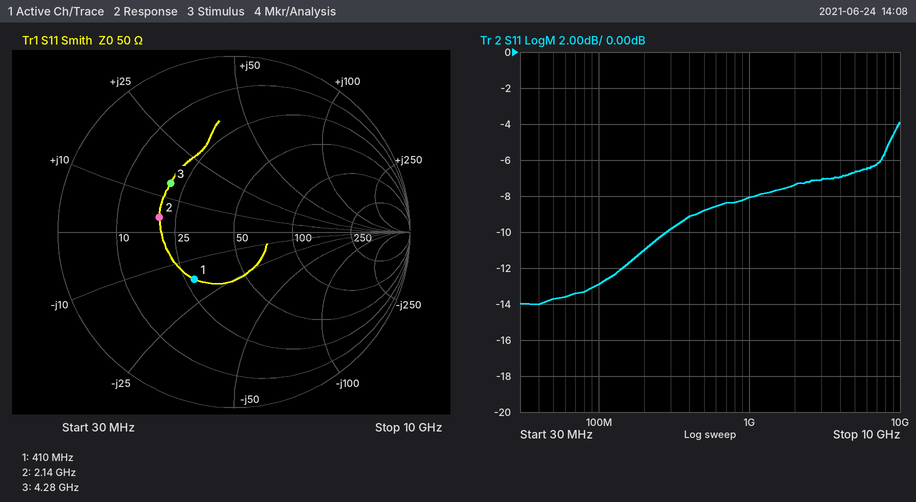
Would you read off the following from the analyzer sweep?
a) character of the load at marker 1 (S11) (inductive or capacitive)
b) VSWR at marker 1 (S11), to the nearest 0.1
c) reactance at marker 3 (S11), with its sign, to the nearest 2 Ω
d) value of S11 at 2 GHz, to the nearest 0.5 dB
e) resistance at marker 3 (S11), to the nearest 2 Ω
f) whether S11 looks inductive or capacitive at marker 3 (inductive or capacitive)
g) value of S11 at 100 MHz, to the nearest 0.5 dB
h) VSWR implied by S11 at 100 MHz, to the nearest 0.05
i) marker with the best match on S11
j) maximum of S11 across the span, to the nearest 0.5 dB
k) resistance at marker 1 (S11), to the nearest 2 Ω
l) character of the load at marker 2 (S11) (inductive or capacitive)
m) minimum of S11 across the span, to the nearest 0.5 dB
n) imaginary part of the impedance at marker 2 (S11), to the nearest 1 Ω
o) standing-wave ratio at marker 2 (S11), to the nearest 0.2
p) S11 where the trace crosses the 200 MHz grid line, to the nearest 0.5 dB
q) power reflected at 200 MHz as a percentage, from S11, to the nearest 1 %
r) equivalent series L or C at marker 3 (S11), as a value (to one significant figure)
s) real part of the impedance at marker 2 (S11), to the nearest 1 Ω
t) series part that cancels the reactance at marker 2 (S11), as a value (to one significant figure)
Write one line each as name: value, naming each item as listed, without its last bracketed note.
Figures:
character of the load at marker 1 (S11): capacitive
VSWR at marker 1 (S11), to the nearest 0.1: 2.1
reactance at marker 3 (S11), with its sign, to the nearest 2 Ω: +14 Ω
value of S11 at 2 GHz, to the nearest 0.5 dB: -7.5 dB
resistance at marker 3 (S11), to the nearest 2 Ω: 20 Ω
whether S11 looks inductive or capacitive at marker 3: inductive
value of S11 at 100 MHz, to the nearest 0.5 dB: -13.0 dB
VSWR implied by S11 at 100 MHz, to the nearest 0.05: 1.60
marker with the best match on S11: marker 1
maximum of S11 across the span, to the nearest 0.5 dB: -4.0 dB
resistance at marker 1 (S11), to the nearest 2 Ω: 28 Ω
character of the load at marker 2 (S11): inductive
minimum of S11 across the span, to the nearest 0.5 dB: -14.0 dB
imaginary part of the impedance at marker 2 (S11), to the nearest 1 Ω: +4 Ω
standing-wave ratio at marker 2 (S11), to the nearest 0.2: 2.6
S11 where the trace crosses the 200 MHz grid line, to the nearest 0.5 dB: -11.0 dB
power reflected at 200 MHz as a percentage, from S11, to the nearest 1 %: 8 %
equivalent series L or C at marker 3 (S11), as a value: 500 pH
real part of the impedance at marker 2 (S11), to the nearest 1 Ω: 20 Ω
series part that cancels the reactance at marker 2 (S11), as a value: 20 pF
